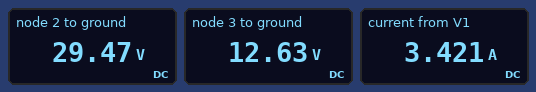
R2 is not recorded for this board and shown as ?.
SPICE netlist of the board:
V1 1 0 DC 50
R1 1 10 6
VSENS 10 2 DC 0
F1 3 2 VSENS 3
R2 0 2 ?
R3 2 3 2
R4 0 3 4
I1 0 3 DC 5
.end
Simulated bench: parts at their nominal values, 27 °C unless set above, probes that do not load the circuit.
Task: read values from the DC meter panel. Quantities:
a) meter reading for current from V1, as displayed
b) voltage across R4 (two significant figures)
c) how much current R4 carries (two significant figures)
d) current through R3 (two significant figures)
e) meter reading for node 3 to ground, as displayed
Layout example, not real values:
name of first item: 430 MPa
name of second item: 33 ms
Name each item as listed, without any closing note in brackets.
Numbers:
meter reading for current from V1, as displayed: 3.421 A
voltage across R4: 13 V
how much current R4 carries: 3.2 A
current through R3: 8.4 A
meter reading for node 3 to ground, as displayed: 12.63 V
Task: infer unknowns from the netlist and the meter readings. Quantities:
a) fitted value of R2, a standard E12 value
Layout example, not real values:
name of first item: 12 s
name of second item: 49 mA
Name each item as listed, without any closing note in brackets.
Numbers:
fitted value of R2, a standard E12 value: 5.6 Ω
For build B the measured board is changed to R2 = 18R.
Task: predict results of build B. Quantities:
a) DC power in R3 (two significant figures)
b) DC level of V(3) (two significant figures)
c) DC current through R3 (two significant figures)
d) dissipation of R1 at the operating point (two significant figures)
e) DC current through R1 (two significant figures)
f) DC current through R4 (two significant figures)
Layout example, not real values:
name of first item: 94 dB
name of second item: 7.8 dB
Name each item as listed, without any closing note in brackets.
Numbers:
DC power in R3: 110 W
DC level of V(3): 21 V
DC current through R3: 7.3 A
dissipation of R1 at the operating point: 33 W
DC current through R1: 2.3 A
DC current through R4: 5.3 A
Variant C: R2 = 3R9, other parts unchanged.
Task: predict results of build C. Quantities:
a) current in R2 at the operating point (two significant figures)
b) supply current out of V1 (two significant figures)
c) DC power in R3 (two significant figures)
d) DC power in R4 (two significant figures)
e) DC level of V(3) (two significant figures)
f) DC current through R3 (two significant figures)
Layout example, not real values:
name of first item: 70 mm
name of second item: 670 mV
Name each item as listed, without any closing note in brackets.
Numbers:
current in R2 at the operating point: 6.8 A
supply current out of V1: 3.9 A
DC power in R3: 160 W
DC power in R4: 18 W
DC level of V(3): 8.6 V
DC current through R3: 8.9 A
